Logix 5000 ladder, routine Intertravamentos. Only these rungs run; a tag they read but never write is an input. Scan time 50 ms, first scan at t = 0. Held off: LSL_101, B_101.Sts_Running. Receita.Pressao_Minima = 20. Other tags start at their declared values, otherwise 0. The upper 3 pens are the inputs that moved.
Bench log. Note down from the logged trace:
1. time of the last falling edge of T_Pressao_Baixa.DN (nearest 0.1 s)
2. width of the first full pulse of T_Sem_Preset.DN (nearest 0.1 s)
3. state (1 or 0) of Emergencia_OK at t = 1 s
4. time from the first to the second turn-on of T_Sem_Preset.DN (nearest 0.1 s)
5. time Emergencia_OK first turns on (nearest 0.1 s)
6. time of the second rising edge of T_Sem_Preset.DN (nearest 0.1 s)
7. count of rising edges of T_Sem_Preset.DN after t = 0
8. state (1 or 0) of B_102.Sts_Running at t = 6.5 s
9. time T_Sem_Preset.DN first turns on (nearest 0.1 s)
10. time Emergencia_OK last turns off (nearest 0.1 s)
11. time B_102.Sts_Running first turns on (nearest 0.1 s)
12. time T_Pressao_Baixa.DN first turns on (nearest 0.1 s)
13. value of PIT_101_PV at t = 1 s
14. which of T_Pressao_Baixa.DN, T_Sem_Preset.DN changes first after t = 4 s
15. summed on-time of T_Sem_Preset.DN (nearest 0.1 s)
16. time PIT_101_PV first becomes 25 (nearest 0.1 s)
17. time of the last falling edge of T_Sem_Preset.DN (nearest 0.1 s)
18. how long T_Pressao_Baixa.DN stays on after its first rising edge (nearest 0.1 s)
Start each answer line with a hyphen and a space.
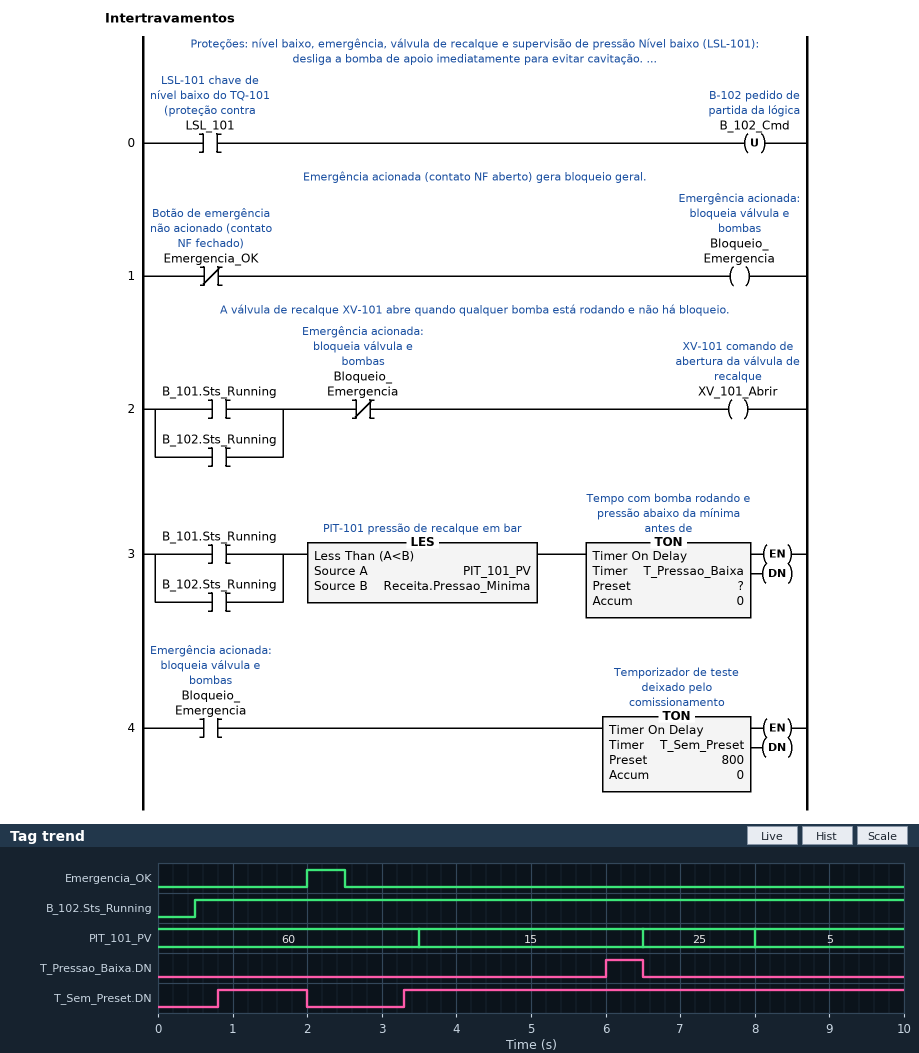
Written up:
- 6.5 s
- 1.2 s
- 0
- 2.5 s
- 2.0 s
- 3.3 s
- 2
- 1
- 0.8 s
- 2.5 s
- 0.5 s
- 6.0 s
- 60
- T_Pressao_Baixa.DN
- 7.9 s
- 6.5 s
- 2.0 s
- 0.5 s
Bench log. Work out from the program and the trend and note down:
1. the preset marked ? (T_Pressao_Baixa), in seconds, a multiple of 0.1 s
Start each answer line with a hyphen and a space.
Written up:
- 2.5 s
